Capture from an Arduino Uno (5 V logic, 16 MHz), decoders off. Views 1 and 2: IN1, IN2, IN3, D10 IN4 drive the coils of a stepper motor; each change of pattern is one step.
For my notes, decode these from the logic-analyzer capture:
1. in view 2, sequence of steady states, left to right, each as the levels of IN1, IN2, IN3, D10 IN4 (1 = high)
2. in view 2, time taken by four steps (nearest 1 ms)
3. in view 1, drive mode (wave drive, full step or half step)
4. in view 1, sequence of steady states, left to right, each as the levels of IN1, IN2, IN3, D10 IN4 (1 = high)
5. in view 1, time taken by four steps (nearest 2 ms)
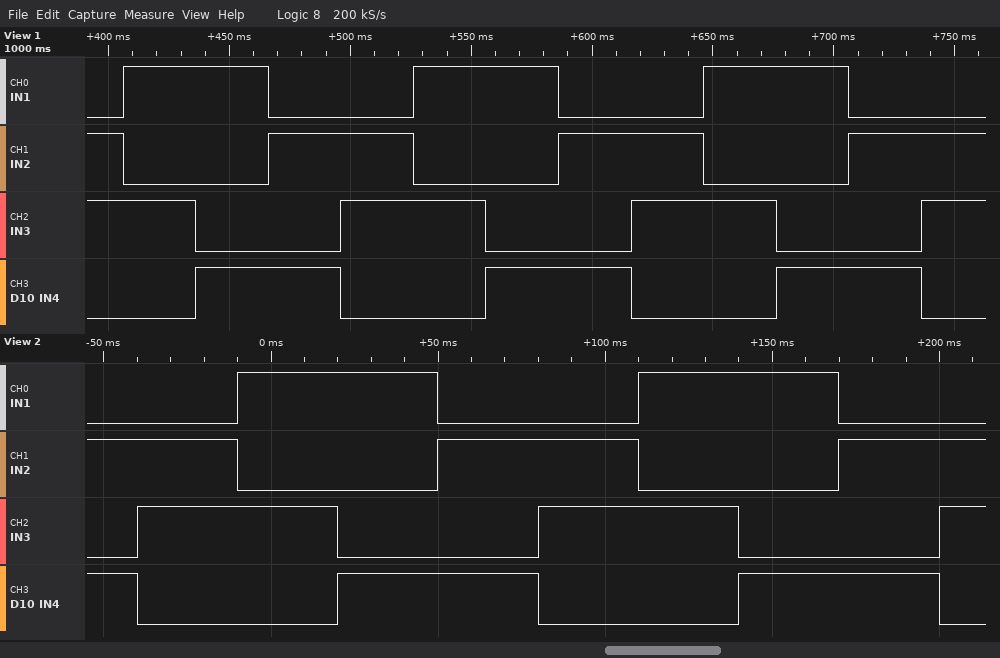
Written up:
0101 0110 1010 1001 0101 0110 1010 1001 0101 0110
120 ms
full step
0110 1010 1001 0101 0110 1010 1001 0101 0110 1010 1001 0101 0110
120 ms
